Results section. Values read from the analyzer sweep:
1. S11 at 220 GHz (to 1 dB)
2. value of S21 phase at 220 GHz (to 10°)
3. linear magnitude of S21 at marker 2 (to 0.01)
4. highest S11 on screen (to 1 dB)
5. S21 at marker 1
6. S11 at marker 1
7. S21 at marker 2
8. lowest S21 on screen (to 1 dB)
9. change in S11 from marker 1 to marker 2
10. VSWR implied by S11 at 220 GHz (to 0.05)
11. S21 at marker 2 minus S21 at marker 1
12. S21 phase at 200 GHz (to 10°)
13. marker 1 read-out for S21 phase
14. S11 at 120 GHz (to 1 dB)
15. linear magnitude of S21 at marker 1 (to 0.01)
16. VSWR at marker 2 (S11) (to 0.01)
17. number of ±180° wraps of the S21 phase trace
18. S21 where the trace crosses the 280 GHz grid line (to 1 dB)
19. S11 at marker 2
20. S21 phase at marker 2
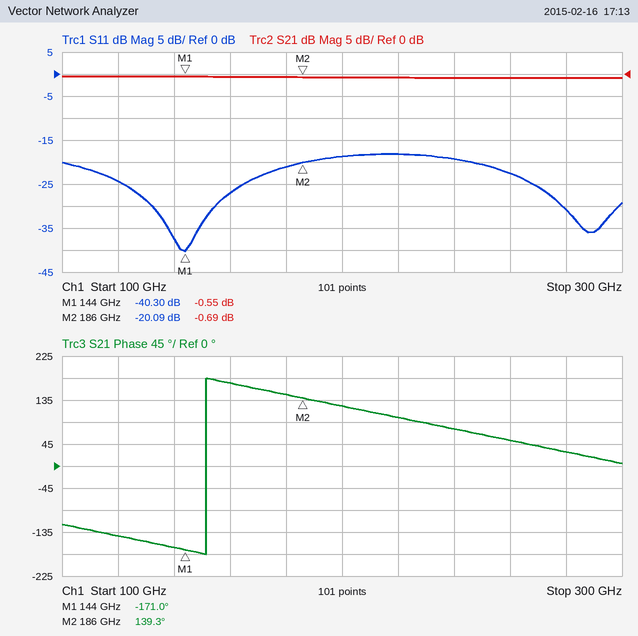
-18 dB
100°
0.92
-18 dB
-0.55 dB
-40.30 dB
-0.69 dB
-1 dB
20.21 dB
1.30
-0.14 dB
120°
-171.0°
-24 dB
0.94
1.22
1
-1 dB
-20.09 dB
139.3°
